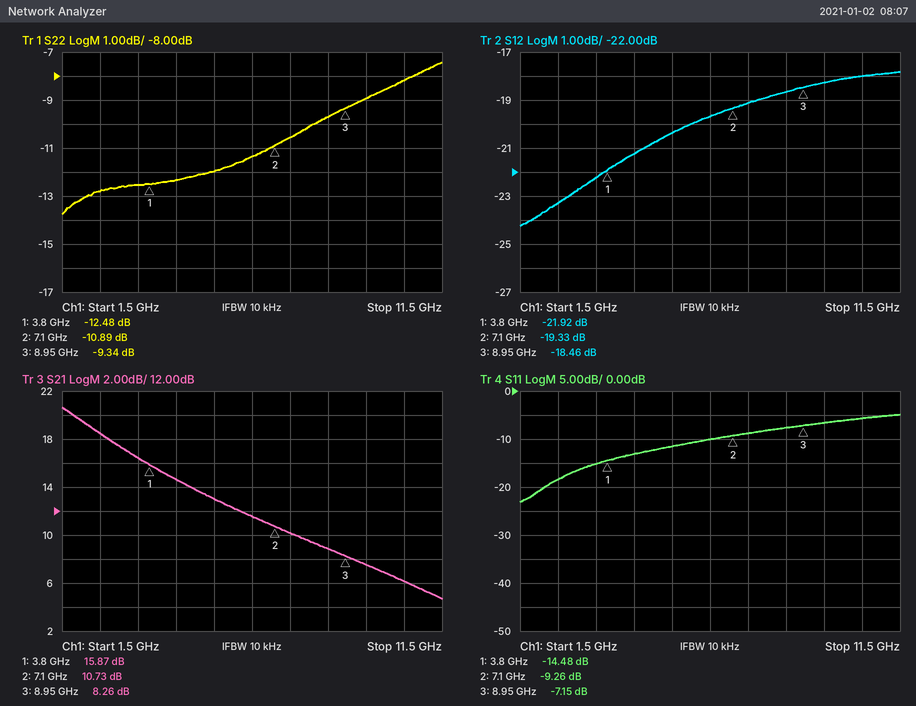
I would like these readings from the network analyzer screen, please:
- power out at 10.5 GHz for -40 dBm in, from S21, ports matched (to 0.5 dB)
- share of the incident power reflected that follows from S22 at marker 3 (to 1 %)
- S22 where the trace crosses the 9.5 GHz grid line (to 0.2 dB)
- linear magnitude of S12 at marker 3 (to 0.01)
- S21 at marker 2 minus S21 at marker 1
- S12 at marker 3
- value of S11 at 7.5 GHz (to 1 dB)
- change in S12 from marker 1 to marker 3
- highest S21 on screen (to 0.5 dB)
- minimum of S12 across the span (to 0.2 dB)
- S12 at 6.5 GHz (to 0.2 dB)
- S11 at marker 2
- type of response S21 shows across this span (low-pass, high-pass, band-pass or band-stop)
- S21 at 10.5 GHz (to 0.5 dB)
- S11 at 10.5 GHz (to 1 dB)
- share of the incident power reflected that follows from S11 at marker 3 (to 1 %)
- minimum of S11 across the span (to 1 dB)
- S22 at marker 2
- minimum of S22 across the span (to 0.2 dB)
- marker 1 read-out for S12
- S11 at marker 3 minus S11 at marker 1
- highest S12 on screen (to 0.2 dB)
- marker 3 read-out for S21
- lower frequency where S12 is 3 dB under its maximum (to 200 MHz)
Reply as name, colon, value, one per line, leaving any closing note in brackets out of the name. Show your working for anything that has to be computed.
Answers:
power out at 10.5 GHz for -40 dBm in, from S21, ports matched: -40 dBm + (6.0 dB) = -34.0 dBm
share of the incident power reflected that follows from S22 at marker 3: 10^(-9.34/10) ≈ 12 %
S22 where the trace crosses the 9.5 GHz grid line: -9.0 dB
linear magnitude of S12 at marker 3: 10^(-18.46/20) ≈ 0.12
S21 at marker 2 minus S21 at marker 1: 10.73 − (15.87) = -5.14 dB
S12 at marker 3: -18.46 dB
value of S11 at 7.5 GHz: -9 dB
change in S12 from marker 1 to marker 3: -18.46 − (-21.92) = 3.46 dB
highest S21 on screen: 20.5 dB
minimum of S12 across the span: -24.2 dB
S12 at 6.5 GHz: -19.6 dB
S11 at marker 2: -9.26 dB
type of response S21 shows across this span: low-pass
S21 at 10.5 GHz: 6.0 dB
S11 at 10.5 GHz: -6 dB
share of the incident power reflected that follows from S11 at marker 3: 10^(-7.15/10) ≈ 19 %
minimum of S11 across the span: -23 dB
S22 at marker 2: -10.89 dB
minimum of S22 across the span: -13.8 dB
marker 1 read-out for S12: -21.92 dB
S11 at marker 3 minus S11 at marker 1: -7.15 − (-14.48) = 7.33 dB
highest S12 on screen: -17.8 dB
marker 3 read-out for S21: 8.26 dB
lower frequency where S12 is 3 dB under its maximum: 5.0 GHz
